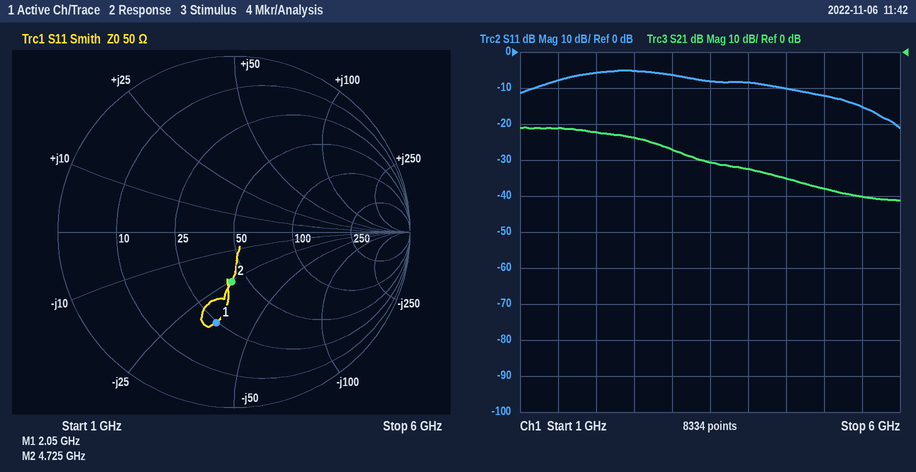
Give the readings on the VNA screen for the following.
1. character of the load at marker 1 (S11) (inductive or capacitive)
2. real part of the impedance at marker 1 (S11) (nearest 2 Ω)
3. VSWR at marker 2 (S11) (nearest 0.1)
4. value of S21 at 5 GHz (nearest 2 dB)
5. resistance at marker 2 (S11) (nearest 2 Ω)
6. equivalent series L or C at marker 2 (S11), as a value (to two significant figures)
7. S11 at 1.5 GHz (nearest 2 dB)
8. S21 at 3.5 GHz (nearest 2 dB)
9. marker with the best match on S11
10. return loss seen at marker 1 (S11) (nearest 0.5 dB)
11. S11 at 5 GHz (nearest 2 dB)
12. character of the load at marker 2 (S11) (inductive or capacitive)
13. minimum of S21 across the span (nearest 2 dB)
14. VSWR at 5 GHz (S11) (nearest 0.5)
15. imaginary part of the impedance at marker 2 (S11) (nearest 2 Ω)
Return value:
capacitive
24 Ω
1.8
-38 dB
42 Ω
1.3 pF
-8 dB
-30 dB
marker 2
5.5 dB
-12 dB
capacitive
-42 dB
1.5
-26 Ω
